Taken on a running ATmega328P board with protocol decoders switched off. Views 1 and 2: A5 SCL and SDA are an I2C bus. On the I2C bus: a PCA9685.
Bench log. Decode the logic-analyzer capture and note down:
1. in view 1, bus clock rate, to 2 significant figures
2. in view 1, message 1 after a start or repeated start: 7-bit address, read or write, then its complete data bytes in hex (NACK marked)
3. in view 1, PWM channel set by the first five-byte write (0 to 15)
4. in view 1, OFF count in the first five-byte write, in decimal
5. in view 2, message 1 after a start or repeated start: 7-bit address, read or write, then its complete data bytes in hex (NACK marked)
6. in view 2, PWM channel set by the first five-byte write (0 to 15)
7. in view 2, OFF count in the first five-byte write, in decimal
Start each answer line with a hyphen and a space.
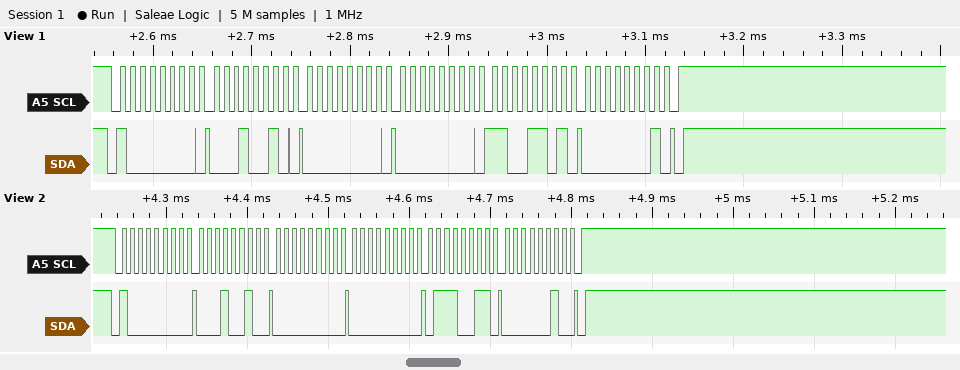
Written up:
- 100 kHz
- 0x40 write: 12 00 00 CD 01
- 3
- 461
- 0x40 write: 12 00 00 73 02
- 3
- 627
